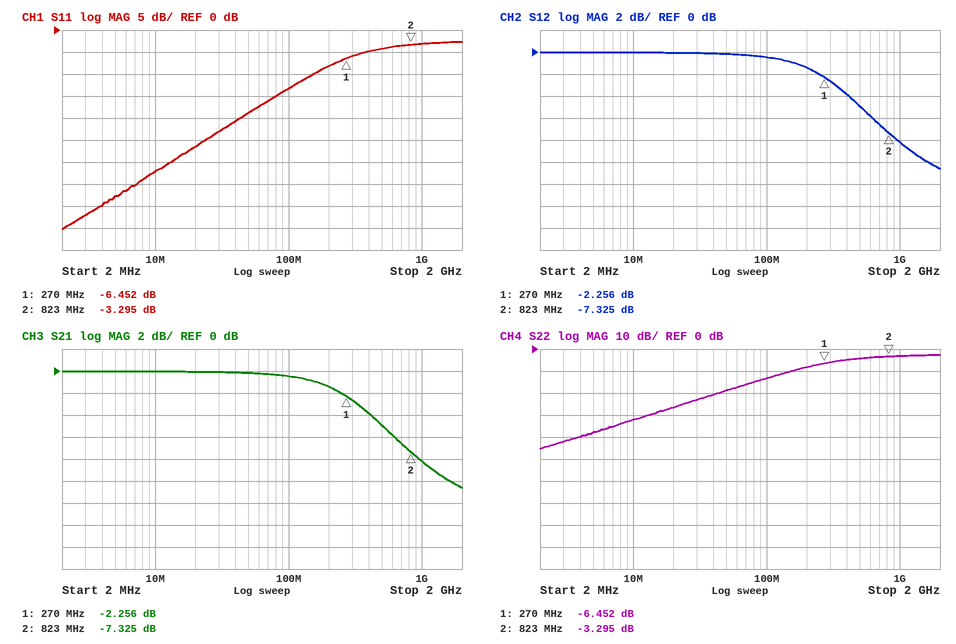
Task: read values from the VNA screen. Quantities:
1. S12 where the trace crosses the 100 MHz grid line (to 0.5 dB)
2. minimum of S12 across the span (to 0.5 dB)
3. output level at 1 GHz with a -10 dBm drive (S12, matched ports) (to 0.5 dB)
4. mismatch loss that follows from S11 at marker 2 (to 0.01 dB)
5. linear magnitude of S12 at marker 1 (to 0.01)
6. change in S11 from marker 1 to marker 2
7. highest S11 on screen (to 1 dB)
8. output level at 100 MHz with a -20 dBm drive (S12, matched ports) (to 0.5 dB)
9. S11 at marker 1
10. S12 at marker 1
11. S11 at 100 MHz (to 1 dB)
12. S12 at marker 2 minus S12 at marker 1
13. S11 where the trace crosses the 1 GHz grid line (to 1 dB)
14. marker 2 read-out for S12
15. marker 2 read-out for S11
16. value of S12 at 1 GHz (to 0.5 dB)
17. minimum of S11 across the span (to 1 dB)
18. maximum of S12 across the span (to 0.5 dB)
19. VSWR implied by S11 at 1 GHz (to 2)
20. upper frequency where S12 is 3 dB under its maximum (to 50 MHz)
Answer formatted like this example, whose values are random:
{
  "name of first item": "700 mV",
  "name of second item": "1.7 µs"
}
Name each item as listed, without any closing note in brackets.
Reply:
{
  "S12 where the trace crosses the 100 MHz grid line": "-0.5 dB",
  "minimum of S12 across the span": "-10.5 dB",
  "output level at 1 GHz with a -10 dBm drive (S12, matched ports)": "-18.0 dBm",
  "mismatch loss that follows from S11 at marker 2": "2.74 dB",
  "linear magnitude of S12 at marker 1": "0.77",
  "change in S11 from marker 1 to marker 2": "3.157 dB",
  "highest S11 on screen": "-3 dB",
  "output level at 100 MHz with a -20 dBm drive (S12, matched ports)": "-20.5 dBm",
  "S11 at marker 1": "-6.452 dB",
  "S12 at marker 1": "-2.256 dB",
  "S11 at 100 MHz": "-13 dB",
  "S12 at marker 2 minus S12 at marker 1": "-5.069 dB",
  "S11 where the trace crosses the 1 GHz grid line": "-3 dB",
  "marker 2 read-out for S12": "-7.325 dB",
  "marker 2 read-out for S11": "-3.295 dB",
  "value of S12 at 1 GHz": "-8.0 dB",
  "minimum of S11 across the span": "-45 dB",
  "maximum of S12 across the span": "0.0 dB",
  "VSWR implied by S11 at 1 GHz": "6",
  "upper frequency where S12 is 3 dB under its maximum": "350 MHz"
}
